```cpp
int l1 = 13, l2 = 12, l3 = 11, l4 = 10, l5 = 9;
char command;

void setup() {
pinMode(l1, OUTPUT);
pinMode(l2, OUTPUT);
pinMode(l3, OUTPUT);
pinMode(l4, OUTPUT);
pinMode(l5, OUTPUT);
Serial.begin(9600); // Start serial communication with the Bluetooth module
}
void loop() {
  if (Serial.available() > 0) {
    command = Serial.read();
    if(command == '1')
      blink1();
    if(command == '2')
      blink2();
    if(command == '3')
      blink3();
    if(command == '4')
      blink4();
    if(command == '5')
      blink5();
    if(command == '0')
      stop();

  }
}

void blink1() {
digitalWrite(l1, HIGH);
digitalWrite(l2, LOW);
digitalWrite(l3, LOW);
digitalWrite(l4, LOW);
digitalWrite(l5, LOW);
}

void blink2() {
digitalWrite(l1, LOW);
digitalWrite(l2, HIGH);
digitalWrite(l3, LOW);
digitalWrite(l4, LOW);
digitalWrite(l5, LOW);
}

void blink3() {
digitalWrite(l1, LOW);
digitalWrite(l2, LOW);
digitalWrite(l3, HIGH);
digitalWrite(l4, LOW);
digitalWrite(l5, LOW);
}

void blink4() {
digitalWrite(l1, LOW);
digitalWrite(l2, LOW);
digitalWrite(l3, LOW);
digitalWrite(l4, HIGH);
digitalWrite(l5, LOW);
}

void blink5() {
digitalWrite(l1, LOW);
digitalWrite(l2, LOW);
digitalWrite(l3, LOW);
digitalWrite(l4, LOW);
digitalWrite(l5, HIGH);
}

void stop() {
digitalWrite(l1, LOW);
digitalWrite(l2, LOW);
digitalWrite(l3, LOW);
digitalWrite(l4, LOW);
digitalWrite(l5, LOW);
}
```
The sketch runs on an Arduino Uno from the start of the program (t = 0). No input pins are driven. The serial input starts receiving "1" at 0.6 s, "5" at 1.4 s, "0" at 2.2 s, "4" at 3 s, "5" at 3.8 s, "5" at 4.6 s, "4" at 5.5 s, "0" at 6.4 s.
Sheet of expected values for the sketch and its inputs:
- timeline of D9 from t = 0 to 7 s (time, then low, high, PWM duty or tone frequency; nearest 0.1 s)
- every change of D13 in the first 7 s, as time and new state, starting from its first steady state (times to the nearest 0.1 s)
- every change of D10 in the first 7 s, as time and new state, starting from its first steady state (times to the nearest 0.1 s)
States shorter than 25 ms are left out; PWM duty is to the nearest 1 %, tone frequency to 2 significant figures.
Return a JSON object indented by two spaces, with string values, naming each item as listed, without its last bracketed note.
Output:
{
  "timeline of D9 from t = 0 to 7 s": "0 s low; 1.4 s high; 2.2 s low; 3.8 s high; 5.5 s low",
  "every change of D13 in the first 7 s, as time and new state, starting from its first steady state": "0 s low; 0.6 s high; 1.4 s low",
  "every change of D10 in the first 7 s, as time and new state, starting from its first steady state": "0 s low; 3 s high; 3.8 s low; 5.5 s high; 6.4 s low"
}
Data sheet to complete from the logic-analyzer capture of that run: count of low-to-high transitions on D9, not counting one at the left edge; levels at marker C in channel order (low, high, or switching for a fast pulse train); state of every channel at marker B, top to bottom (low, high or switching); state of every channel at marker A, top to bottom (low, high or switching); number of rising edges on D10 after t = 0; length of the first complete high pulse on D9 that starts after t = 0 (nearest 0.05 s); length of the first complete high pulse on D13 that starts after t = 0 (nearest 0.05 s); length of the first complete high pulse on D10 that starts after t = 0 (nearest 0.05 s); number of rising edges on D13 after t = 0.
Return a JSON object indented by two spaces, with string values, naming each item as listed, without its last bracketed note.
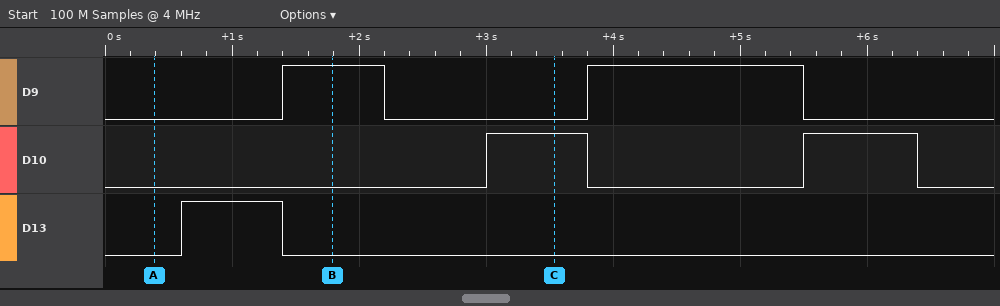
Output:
{
  "count of low-to-high transitions on D9, not counting one at the left edge": "2",
  "levels at marker C in channel order": "D9 low, D10 high, D13 low",
  "state of every channel at marker B, top to bottom": "D9 high, D10 low, D13 low",
  "state of every channel at marker A, top to bottom": "D9 low, D10 low, D13 low",
  "number of rising edges on D10 after t = 0": "2",
  "length of the first complete high pulse on D9 that starts after t = 0": "0.80 s",
  "length of the first complete high pulse on D13 that starts after t = 0": "0.80 s",
  "length of the first complete high pulse on D10 that starts after t = 0": "0.80 s",
  "number of rising edges on D13 after t = 0": "1"
}
